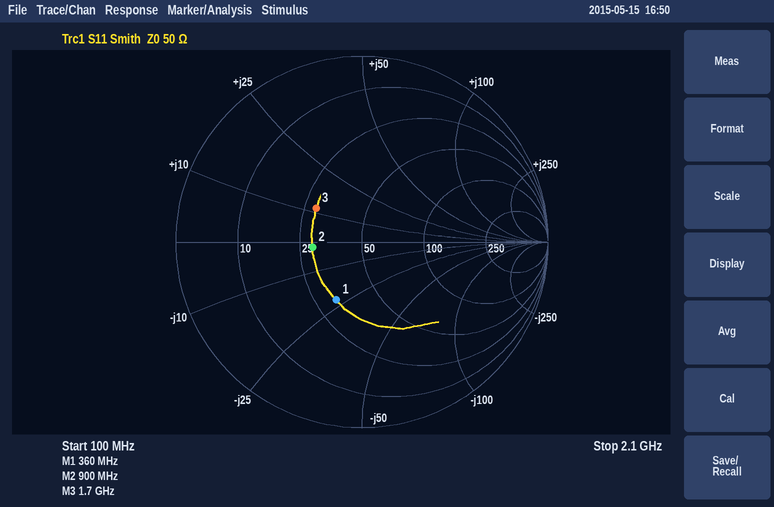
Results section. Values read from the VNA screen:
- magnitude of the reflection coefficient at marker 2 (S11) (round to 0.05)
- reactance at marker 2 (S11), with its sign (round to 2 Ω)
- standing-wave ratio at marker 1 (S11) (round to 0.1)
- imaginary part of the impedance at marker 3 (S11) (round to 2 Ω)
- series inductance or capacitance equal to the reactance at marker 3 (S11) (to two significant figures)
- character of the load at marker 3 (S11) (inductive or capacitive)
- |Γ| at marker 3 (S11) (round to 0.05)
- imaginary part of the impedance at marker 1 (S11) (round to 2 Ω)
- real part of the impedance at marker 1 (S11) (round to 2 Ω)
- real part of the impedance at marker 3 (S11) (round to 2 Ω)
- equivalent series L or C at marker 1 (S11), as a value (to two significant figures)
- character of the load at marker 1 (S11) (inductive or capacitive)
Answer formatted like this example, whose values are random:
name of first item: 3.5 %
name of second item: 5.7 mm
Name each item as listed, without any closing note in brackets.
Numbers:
magnitude of the reflection coefficient at marker 2 (S11): 0.25
reactance at marker 2 (S11), with its sign: -2 Ω
standing-wave ratio at marker 1 (S11): 2.0
imaginary part of the impedance at marker 3 (S11): +12 Ω
series inductance or capacitance equal to the reactance at marker 3 (S11): 1.1 nH
character of the load at marker 3 (S11): inductive
|Γ| at marker 3 (S11): 0.30
imaginary part of the impedance at marker 1 (S11): -22 Ω
real part of the impedance at marker 1 (S11): 32 Ω
real part of the impedance at marker 3 (S11): 28 Ω
equivalent series L or C at marker 1 (S11), as a value: 20 pF
character of the load at marker 1 (S11): capacitive
